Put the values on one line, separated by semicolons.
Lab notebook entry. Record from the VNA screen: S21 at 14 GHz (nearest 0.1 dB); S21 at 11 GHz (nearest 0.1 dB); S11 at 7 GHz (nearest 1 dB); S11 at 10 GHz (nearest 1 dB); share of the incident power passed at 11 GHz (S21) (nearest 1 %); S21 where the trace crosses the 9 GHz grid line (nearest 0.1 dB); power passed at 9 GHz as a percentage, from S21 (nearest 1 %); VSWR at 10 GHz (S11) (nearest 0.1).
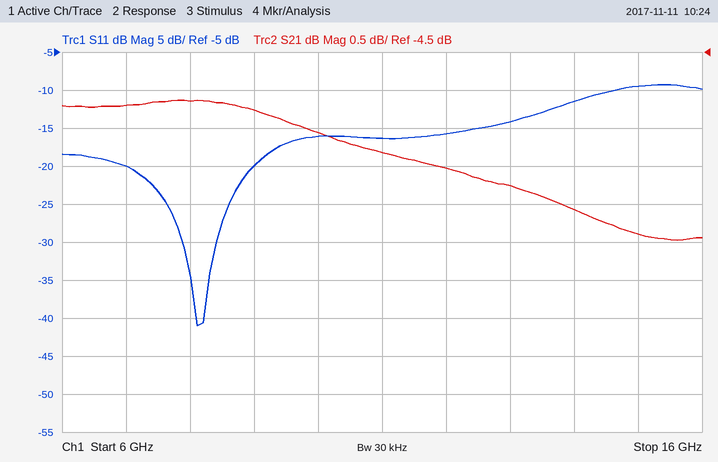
-6.6 dB; -5.8 dB; -20 dB; -16 dB; 26 %; -5.3 dB; 30 %; 1.4
